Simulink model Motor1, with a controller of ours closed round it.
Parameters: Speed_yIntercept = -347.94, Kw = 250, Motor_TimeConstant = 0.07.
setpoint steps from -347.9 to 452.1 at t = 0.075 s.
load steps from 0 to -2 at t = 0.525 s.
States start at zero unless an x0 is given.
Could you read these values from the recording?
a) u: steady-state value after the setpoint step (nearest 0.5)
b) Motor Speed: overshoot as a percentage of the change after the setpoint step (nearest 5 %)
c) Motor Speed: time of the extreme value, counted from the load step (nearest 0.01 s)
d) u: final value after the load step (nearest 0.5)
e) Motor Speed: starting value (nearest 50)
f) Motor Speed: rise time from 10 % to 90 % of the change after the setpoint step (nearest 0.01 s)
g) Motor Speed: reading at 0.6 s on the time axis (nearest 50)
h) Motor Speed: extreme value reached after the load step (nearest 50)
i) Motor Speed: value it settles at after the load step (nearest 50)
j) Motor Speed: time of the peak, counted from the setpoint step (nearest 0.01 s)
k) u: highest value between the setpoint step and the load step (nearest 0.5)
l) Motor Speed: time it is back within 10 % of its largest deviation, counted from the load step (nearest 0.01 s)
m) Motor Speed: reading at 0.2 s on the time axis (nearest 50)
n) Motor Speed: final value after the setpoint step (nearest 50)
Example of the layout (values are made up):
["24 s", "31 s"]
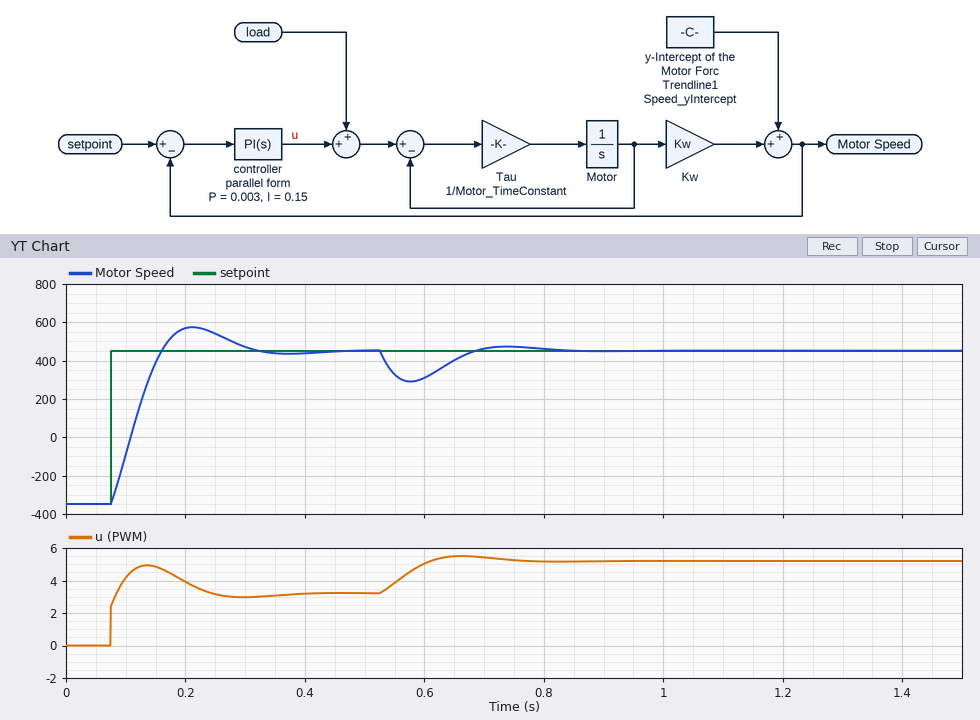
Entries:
["3.0", "15 %", "0.05 s", "5.0", "-350", "0.06 s", "300", "300", "450", "0.14 s", "5.0", "0.25 s", "550", "450"]
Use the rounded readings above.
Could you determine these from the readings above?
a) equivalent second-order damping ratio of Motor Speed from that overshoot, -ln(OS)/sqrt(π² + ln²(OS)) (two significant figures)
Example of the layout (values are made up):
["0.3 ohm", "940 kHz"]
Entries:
["0.52"]
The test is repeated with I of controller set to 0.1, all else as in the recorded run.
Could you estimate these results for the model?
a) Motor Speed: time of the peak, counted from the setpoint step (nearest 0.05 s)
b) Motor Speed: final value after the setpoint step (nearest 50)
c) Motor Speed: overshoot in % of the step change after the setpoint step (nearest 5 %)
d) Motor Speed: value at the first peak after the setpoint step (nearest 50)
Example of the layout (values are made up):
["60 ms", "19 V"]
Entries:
["0.20 s", "450", "10 %", "500"]
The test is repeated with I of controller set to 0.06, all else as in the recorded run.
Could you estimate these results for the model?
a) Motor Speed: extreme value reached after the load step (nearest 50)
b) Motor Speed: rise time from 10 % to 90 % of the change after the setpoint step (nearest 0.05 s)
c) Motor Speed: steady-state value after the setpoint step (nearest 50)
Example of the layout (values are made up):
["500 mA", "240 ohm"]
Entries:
["250", "0.15 s", "450"]
